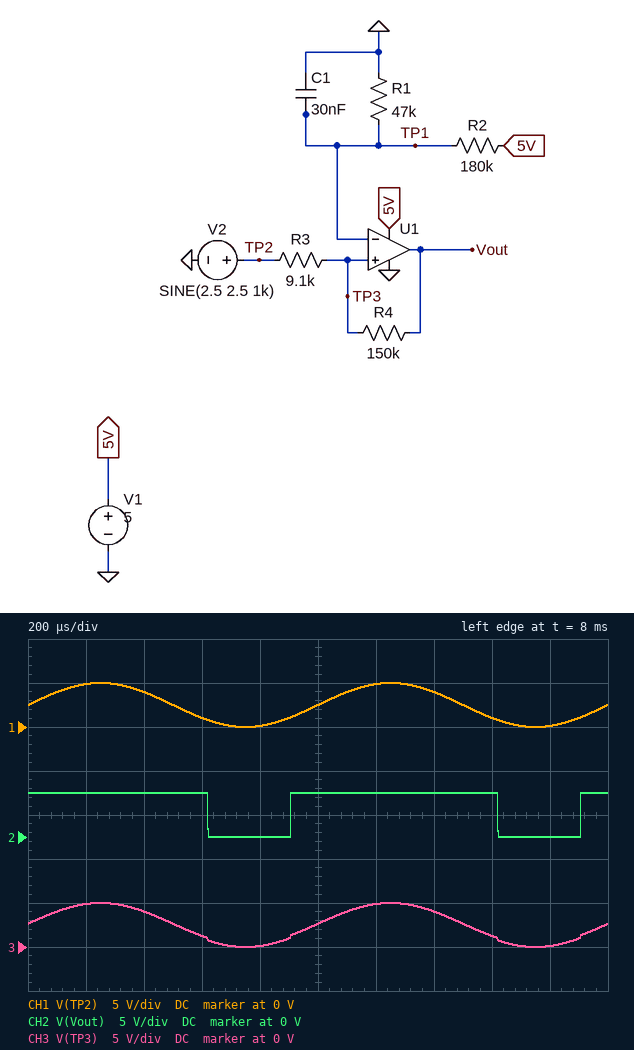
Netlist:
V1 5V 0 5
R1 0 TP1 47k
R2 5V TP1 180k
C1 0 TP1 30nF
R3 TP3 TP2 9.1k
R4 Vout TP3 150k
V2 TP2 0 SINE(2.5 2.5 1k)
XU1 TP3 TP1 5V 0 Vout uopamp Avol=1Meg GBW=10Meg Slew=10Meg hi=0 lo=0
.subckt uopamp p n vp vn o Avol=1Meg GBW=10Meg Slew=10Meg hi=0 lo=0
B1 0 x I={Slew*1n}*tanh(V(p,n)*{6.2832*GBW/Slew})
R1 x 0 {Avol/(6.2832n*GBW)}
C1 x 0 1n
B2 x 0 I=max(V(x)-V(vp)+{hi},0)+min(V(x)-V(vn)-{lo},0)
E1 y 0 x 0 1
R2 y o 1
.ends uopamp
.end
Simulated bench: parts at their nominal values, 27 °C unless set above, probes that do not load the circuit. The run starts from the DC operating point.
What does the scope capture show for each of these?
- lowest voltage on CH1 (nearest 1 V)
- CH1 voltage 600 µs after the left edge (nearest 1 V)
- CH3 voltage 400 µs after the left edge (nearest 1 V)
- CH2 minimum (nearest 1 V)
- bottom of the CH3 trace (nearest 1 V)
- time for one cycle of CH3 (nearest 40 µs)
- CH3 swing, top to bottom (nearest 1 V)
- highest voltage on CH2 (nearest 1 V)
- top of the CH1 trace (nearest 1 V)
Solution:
0 V
1 V
4 V
0 V
0 V
1.00 ms
5 V
5 V
5 V
